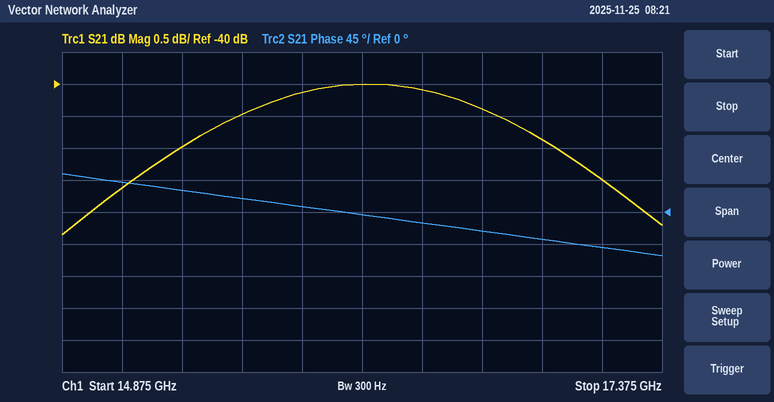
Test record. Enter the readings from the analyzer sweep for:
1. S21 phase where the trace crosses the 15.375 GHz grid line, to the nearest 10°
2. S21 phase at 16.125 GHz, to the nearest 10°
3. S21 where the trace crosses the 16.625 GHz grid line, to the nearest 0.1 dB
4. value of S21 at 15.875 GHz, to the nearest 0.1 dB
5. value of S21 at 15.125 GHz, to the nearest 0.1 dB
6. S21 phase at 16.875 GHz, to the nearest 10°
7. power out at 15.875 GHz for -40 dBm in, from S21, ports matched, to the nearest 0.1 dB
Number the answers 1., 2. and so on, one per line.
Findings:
1. 30°
2. 0°
3. -40.4 dB
4. -40.1 dB
5. -41.6 dB
6. -40°
7. -80.1 dBm
